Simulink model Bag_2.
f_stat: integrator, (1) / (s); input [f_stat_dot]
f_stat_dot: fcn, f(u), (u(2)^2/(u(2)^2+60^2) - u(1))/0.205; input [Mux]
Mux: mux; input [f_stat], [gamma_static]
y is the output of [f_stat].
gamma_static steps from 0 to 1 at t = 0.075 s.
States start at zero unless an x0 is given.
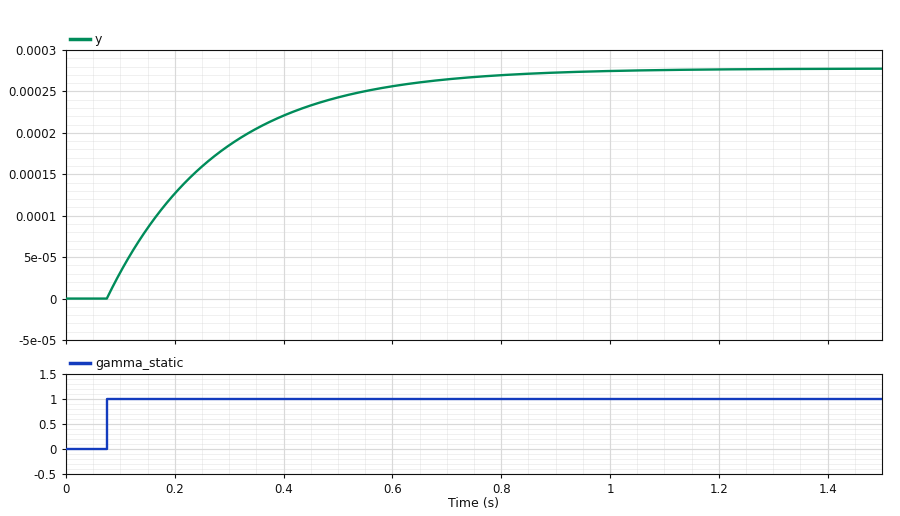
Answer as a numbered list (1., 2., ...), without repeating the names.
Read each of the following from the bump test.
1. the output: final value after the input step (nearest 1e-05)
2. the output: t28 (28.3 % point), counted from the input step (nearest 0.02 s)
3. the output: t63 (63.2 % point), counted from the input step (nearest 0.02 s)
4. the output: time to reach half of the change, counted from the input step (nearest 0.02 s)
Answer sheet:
1. 0.00028
2. 0.06 s
3. 0.20 s
4. 0.14 s
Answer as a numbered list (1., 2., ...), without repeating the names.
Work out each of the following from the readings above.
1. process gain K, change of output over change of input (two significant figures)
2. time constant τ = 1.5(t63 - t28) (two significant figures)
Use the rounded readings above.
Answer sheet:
1. 0.00028
2. 0.21 s
